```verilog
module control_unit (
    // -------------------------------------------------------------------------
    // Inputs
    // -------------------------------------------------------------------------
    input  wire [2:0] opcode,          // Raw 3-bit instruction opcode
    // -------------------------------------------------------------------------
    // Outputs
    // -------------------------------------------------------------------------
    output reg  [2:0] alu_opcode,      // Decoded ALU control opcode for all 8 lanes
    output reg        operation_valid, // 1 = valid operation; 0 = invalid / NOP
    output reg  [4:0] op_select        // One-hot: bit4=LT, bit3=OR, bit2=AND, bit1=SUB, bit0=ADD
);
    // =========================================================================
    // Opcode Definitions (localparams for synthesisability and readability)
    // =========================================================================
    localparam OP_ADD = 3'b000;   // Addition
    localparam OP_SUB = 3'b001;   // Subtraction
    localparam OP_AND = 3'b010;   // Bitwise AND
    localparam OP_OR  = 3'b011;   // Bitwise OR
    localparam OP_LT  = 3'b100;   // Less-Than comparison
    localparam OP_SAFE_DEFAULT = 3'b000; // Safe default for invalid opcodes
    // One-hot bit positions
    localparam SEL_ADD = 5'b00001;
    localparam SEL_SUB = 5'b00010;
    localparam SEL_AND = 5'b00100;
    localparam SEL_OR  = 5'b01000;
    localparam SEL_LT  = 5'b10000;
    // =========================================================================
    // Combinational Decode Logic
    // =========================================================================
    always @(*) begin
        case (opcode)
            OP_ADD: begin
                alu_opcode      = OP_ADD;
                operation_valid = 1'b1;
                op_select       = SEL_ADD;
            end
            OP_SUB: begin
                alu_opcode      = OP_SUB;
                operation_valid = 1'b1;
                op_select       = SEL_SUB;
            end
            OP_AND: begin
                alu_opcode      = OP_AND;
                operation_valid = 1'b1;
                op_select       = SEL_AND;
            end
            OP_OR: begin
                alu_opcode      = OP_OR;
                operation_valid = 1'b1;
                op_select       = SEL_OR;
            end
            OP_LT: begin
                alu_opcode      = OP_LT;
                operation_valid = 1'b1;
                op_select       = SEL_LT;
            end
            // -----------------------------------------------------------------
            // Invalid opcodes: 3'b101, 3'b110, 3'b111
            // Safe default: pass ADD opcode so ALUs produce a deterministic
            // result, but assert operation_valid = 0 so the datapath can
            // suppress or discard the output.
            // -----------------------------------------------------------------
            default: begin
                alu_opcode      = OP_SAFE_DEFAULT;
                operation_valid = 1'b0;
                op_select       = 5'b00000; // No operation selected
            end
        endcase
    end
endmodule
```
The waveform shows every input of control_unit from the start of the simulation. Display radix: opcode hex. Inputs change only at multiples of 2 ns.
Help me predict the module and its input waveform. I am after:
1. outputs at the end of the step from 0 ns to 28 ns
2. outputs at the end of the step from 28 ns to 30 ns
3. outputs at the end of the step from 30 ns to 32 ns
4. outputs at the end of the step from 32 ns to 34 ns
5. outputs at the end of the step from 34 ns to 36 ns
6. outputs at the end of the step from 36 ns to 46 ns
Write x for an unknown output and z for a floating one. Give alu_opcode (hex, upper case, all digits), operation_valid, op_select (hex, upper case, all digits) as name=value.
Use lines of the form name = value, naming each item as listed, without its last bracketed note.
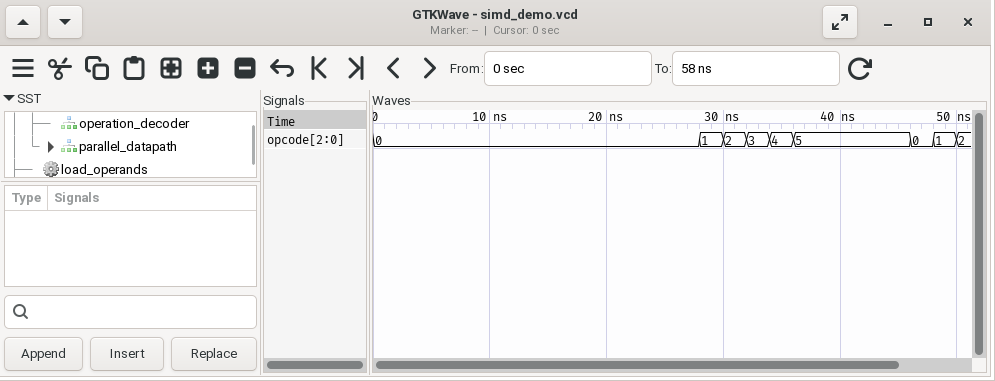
outputs at the end of the step from 0 ns to 28 ns = alu_opcode=0, operation_valid=1, op_select=01
outputs at the end of the step from 28 ns to 30 ns = alu_opcode=1, operation_valid=1, op_select=02
outputs at the end of the step from 30 ns to 32 ns = alu_opcode=2, operation_valid=1, op_select=04
outputs at the end of the step from 32 ns to 34 ns = alu_opcode=3, operation_valid=1, op_select=08
outputs at the end of the step from 34 ns to 36 ns = alu_opcode=4, operation_valid=1, op_select=10
outputs at the end of the step from 36 ns to 46 ns = alu_opcode=0, operation_valid=0, op_select=00
